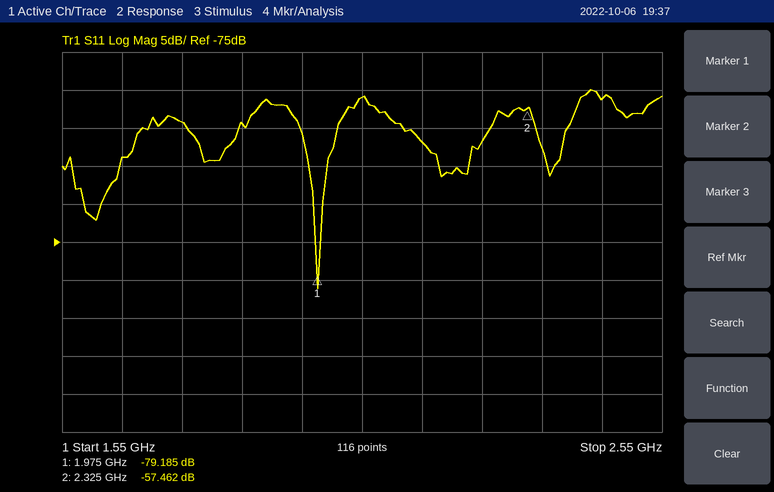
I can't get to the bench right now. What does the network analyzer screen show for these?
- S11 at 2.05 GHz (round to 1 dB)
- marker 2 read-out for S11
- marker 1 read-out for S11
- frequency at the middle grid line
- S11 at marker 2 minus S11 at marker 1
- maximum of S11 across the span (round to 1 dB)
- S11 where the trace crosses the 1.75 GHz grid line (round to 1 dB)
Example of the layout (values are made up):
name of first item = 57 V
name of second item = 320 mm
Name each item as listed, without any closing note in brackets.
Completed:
S11 at 2.05 GHz = -56 dB
marker 2 read-out for S11 = -57.462 dB
marker 1 read-out for S11 = -79.185 dB
frequency at the middle grid line = 2.05 GHz
S11 at marker 2 minus S11 at marker 1 = 21.723 dB
maximum of S11 across the span = -55 dB
S11 where the trace crosses the 1.75 GHz grid line = -59 dB
